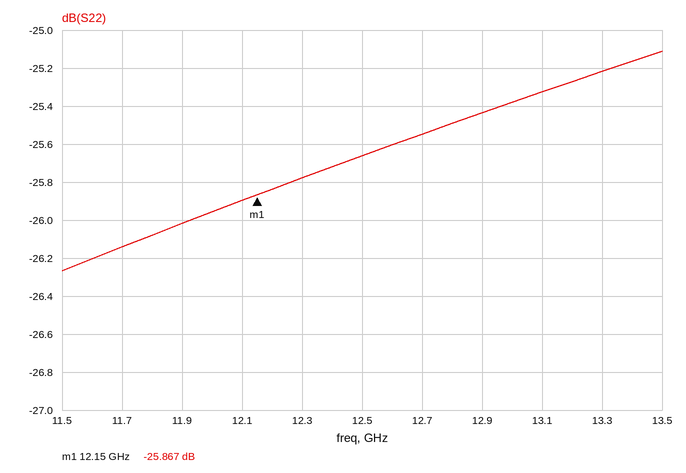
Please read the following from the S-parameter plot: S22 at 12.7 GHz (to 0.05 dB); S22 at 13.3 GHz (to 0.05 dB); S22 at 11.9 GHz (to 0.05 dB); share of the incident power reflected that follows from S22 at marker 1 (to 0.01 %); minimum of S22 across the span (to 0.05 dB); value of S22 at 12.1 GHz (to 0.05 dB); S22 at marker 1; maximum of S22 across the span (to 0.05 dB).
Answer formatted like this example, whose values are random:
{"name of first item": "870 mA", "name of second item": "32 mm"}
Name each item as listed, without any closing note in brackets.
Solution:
{"S22 at 12.7 GHz": "-25.55 dB", "S22 at 13.3 GHz": "-25.20 dB", "S22 at 11.9 GHz": "-26.00 dB", "share of the incident power reflected that follows from S22 at marker 1": "0.26 %", "minimum of S22 across the span": "-26.25 dB", "value of S22 at 12.1 GHz": "-25.90 dB", "S22 at marker 1": "-25.867 dB", "maximum of S22 across the span": "-25.10 dB"}
